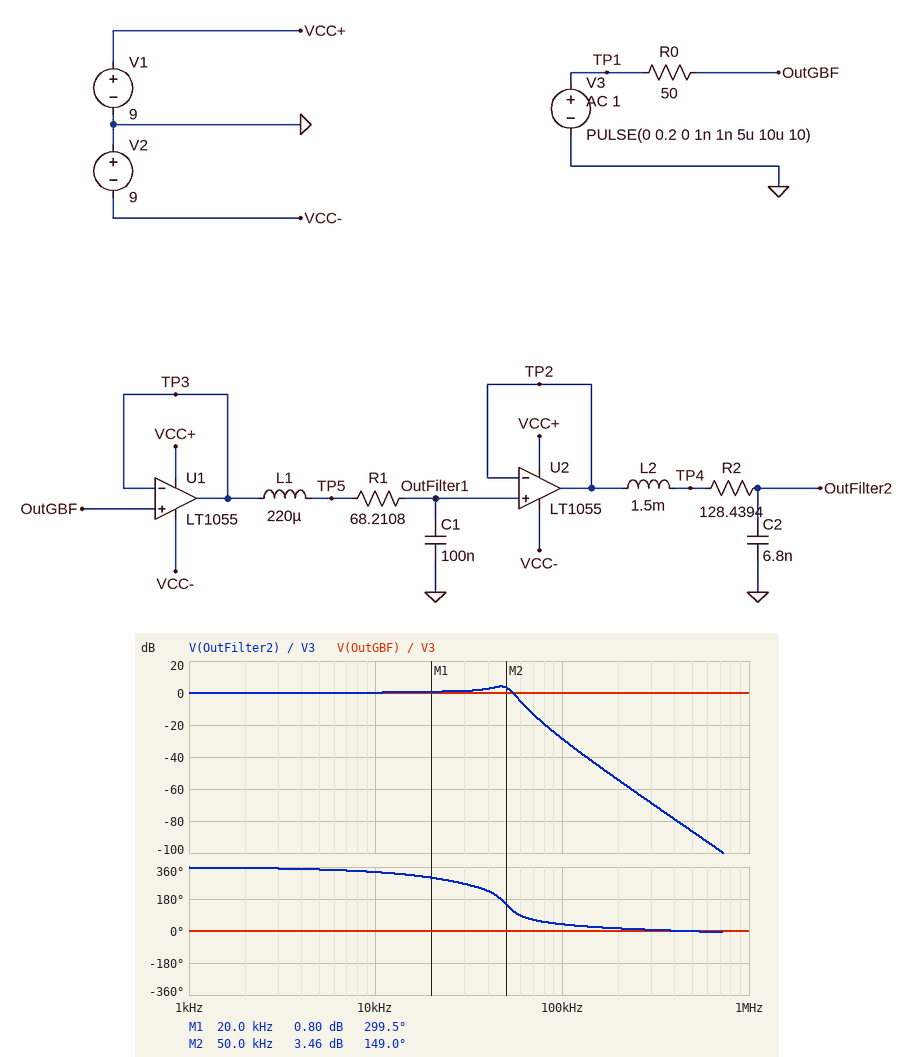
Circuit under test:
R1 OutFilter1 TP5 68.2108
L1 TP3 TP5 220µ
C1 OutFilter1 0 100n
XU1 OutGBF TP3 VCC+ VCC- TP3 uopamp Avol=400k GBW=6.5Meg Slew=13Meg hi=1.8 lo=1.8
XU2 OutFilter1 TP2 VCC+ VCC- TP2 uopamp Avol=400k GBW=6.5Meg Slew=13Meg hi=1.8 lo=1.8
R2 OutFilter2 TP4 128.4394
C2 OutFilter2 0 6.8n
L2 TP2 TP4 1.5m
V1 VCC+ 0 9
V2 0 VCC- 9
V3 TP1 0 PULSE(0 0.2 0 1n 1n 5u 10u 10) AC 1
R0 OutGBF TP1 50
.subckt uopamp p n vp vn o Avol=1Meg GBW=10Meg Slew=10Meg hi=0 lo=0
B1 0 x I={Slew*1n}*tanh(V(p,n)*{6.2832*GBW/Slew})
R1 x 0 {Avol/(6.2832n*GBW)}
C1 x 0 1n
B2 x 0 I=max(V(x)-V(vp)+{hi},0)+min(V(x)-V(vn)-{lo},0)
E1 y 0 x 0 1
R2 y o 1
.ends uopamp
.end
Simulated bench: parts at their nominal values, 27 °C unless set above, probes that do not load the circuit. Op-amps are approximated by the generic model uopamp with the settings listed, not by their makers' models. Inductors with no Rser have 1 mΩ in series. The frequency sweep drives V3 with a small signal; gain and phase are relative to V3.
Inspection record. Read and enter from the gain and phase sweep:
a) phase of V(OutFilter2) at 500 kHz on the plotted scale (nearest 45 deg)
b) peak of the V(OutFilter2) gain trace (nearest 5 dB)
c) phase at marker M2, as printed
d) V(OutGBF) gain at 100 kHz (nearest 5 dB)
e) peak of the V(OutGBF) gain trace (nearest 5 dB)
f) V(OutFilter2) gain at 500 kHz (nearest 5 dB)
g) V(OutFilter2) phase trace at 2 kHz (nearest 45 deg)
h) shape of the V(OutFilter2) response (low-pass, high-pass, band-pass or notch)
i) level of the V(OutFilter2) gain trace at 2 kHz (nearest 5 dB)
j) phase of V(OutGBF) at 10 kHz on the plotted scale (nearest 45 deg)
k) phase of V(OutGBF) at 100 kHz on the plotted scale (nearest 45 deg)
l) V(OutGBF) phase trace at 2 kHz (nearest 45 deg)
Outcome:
0 deg
5 dB
149.0 deg
0 dB
0 dB
-85 dB
360 deg
low-pass
0 dB
0 deg
0 deg
0 deg
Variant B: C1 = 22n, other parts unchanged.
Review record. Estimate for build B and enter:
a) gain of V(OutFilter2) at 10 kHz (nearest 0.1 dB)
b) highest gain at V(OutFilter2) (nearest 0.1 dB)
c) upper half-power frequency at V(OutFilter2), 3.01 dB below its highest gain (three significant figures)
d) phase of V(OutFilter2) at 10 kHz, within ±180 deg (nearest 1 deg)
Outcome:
0.5 dB
14.3 dB
56.2 kHz
-9 deg
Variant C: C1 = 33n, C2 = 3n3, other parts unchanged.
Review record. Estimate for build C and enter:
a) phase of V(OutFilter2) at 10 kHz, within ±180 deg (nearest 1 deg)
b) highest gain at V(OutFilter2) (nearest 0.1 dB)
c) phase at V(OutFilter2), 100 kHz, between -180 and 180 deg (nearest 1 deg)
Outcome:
-10 deg
13.8 dB
51 deg
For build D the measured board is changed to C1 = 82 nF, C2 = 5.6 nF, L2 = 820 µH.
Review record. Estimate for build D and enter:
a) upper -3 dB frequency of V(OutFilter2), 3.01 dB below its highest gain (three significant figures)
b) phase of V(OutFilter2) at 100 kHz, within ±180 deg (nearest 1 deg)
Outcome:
74.2 kHz
57 deg
